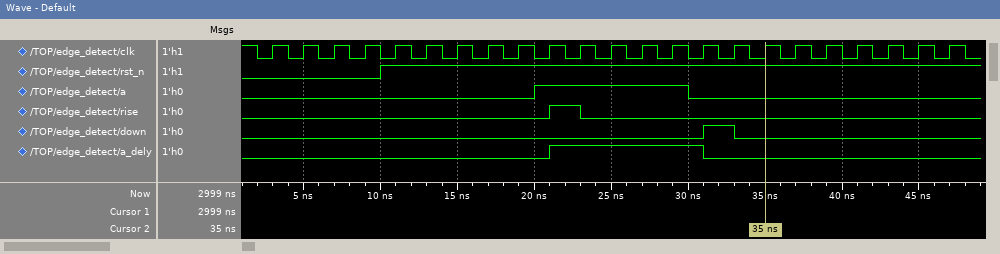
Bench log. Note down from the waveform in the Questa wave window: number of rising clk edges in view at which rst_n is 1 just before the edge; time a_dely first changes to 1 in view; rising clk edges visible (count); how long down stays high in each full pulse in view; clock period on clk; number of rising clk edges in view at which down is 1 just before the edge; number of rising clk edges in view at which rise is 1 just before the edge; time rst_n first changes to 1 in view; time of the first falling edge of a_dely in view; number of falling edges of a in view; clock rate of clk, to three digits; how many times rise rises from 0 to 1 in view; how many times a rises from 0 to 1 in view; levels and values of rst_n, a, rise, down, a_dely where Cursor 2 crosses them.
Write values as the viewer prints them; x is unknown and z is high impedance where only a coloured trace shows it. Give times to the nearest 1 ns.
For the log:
19
21 ns
23
2 ns
2 ns
1
1
10 ns
31 ns
1
500 MHz
1
1
rst_n=1, a=0, rise=0, down=0, a_dely=0
